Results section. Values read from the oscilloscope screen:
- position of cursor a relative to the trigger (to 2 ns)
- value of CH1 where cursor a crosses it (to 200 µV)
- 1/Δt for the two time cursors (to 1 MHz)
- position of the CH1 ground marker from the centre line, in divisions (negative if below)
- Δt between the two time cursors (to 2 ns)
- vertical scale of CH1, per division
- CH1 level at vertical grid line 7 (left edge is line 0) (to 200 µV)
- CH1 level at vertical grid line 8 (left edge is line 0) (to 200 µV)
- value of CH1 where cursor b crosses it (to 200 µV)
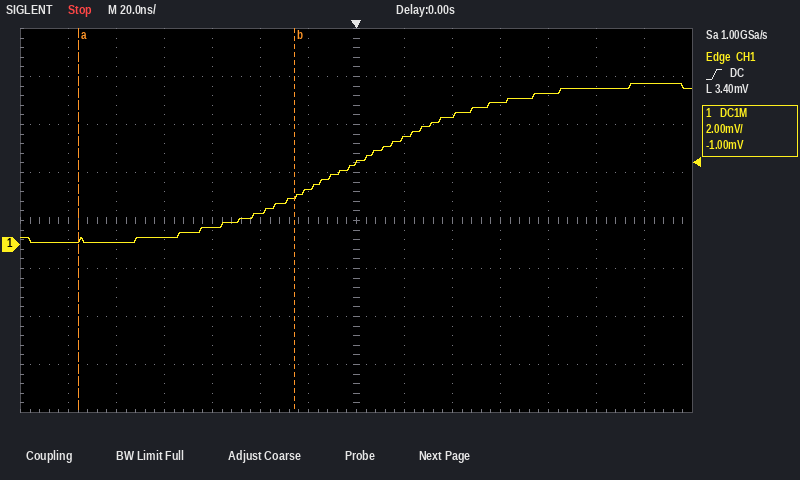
-116 ns
200 µV
11 MHz
-0.5 div
90 ns
2 mV
3.4 mV
4.4 mV
2.0 mV
